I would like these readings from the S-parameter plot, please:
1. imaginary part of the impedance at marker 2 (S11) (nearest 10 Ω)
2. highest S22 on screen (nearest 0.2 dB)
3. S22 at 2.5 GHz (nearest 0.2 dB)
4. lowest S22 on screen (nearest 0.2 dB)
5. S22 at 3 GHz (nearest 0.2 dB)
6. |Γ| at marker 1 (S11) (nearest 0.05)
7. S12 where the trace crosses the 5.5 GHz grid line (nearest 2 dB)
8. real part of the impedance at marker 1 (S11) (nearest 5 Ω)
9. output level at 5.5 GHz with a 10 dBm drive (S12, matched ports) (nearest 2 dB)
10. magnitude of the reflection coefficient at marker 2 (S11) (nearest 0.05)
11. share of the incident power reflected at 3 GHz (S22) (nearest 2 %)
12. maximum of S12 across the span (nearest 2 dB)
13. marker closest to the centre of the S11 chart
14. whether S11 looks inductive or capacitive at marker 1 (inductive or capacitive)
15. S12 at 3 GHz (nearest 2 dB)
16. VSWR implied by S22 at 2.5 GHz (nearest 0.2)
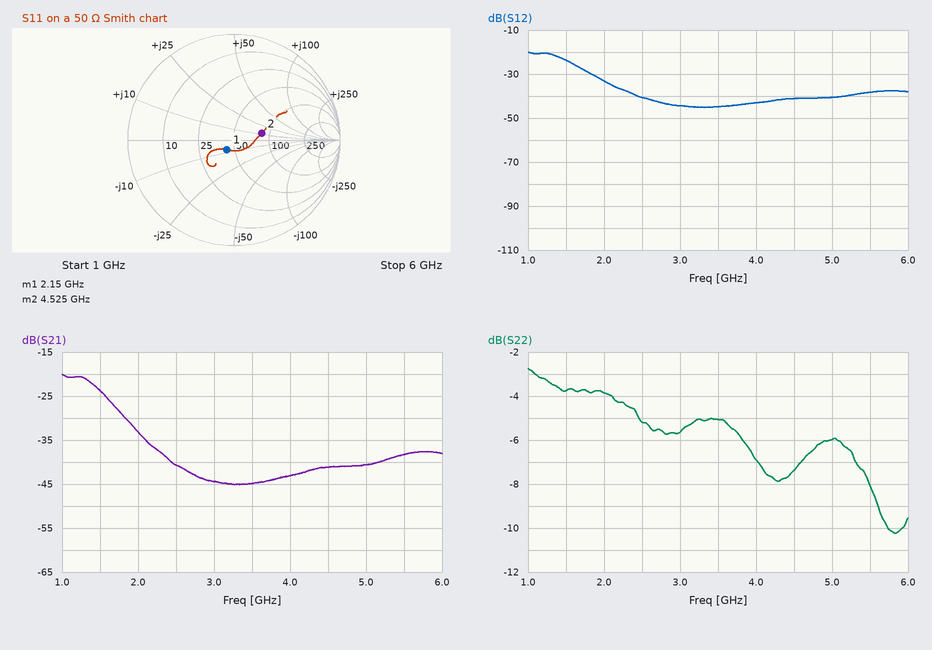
+10 Ω
-2.8 dB
-5.2 dB
-10.2 dB
-5.6 dB
0.10
-38 dB
45 Ω
-28 dBm
0.25
28 %
-20 dB
marker 1
capacitive
-44 dB
3.4
